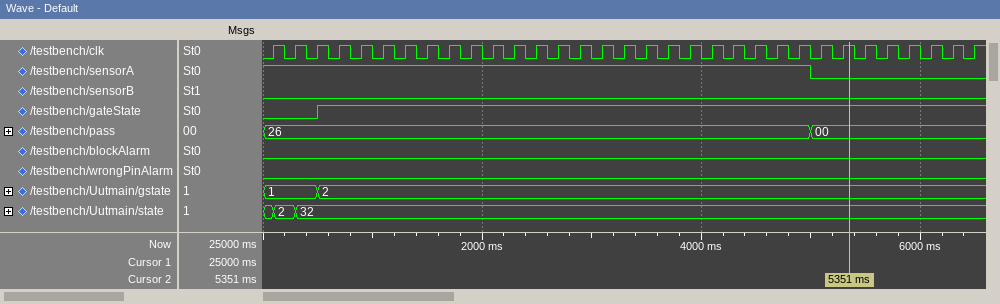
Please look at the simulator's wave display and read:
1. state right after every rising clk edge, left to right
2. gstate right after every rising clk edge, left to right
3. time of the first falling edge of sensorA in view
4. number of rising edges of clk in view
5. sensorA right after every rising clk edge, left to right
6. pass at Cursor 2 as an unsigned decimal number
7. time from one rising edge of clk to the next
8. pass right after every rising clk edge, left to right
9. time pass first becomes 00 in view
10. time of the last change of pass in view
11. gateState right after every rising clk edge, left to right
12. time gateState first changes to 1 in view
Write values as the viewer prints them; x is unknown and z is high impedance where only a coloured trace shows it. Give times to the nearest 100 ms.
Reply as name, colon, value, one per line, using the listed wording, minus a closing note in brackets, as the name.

state right after every rising clk edge, left to right: 2, 32, 32, 32, 32, 32, 32, 32, 32, 32, 32, 32, 32, 32, 32, 32, 32, 32, 32, 32, 32, 32, 32, 32, 32, 32, 32, 32, 32, 32, 32, 32, 32
gstate right after every rising clk edge, left to right: 1, 1, 2, 2, 2, 2, 2, 2, 2, 2, 2, 2, 2, 2, 2, 2, 2, 2, 2, 2, 2, 2, 2, 2, 2, 2, 2, 2, 2, 2, 2, 2, 2
time of the first falling edge of sensorA in view: 5000 ms
number of rising edges of clk in view: 33
sensorA right after every rising clk edge, left to right: 1 1 1 1 1 1 1 1 1 1 1 1 1 1 1 1 1 1 1 1 1 1 1 1 1 0 0 0 0 0 0 0 0
pass at Cursor 2 as an unsigned decimal number: 0
time from one rising edge of clk to the next: 200 ms
pass right after every rising clk edge, left to right: 26, 26, 26, 26, 26, 26, 26, 26, 26, 26, 26, 26, 26, 26, 26, 26, 26, 26, 26, 26, 26, 26, 26, 26, 26, 00, 00, 00, 00, 00, 00, 00, 00
time pass first becomes 00 in view: 5000 ms
time of the last change of pass in view: 5000 ms
gateState right after every rising clk edge, left to right: 0 0 1 1 1 1 1 1 1 1 1 1 1 1 1 1 1 1 1 1 1 1 1 1 1 1 1 1 1 1 1 1 1
time gateState first changes to 1 in view: 500 ms
